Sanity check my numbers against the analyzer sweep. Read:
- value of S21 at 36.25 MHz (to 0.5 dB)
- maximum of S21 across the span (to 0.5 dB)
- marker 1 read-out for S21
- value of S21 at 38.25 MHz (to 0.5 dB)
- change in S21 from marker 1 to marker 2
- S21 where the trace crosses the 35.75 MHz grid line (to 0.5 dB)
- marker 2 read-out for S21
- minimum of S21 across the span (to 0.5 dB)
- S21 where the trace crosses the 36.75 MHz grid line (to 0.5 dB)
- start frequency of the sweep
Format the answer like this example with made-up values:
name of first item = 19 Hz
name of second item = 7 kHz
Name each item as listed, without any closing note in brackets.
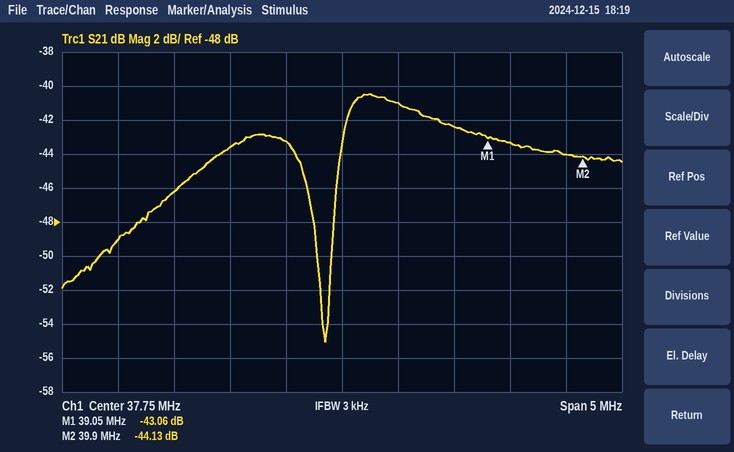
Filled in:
value of S21 at 36.25 MHz = -46.0 dB
maximum of S21 across the span = -40.5 dB
marker 1 read-out for S21 = -43.06 dB
value of S21 at 38.25 MHz = -41.0 dB
change in S21 from marker 1 to marker 2 = -1.07 dB
S21 where the trace crosses the 35.75 MHz grid line = -49.0 dB
marker 2 read-out for S21 = -44.13 dB
minimum of S21 across the span = -55.0 dB
S21 where the trace crosses the 36.75 MHz grid line = -43.5 dB
start frequency of the sweep = 35.25 MHz
